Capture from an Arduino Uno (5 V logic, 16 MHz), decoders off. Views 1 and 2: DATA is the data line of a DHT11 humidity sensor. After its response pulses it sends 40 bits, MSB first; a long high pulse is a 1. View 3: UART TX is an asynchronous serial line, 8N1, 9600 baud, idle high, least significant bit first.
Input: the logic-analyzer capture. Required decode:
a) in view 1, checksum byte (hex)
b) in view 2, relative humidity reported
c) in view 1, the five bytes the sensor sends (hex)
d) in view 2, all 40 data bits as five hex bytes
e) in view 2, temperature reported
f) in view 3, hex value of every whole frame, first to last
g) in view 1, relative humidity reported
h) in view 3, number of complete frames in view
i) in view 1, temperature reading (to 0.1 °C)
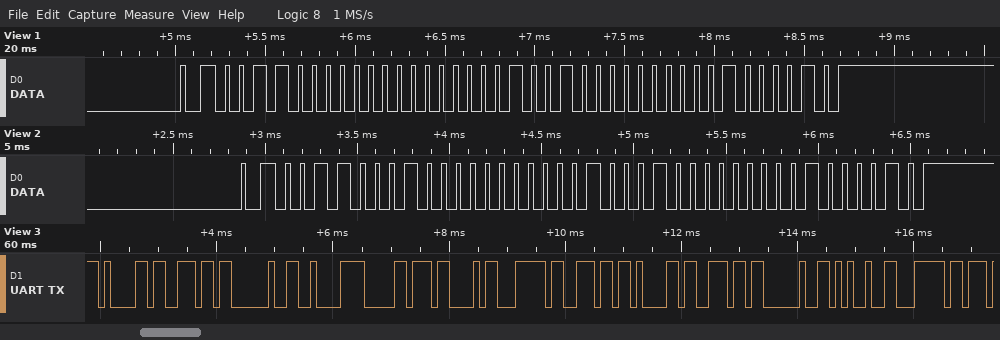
0x42
49 %
30 00 12 00 42
31 00 11 00 42
17.0 °C
61 6E 20 C2 B0 43 7C 6E 61 6E 20 25 7C
48 %
13
18.0 °C
